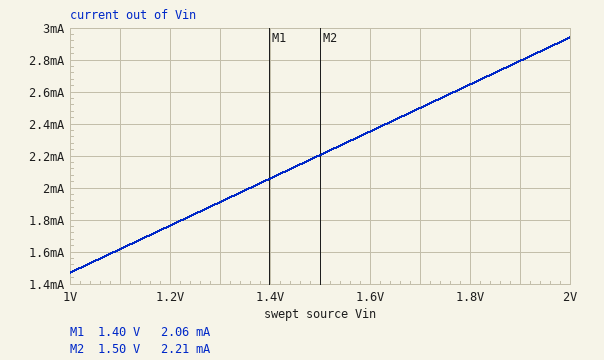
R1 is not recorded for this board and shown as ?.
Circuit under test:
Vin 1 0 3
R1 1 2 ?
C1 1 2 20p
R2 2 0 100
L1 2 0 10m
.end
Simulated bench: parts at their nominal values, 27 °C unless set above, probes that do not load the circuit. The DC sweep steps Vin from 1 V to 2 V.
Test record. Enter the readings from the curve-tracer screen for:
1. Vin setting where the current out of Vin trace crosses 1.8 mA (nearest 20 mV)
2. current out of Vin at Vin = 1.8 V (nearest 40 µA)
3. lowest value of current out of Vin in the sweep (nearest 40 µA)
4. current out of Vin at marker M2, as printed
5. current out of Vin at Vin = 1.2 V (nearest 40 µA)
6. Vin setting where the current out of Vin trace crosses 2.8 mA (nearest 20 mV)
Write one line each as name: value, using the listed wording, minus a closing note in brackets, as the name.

Vin setting where the current out of Vin trace crosses 1.8 mA: 1.22 V
current out of Vin at Vin = 1.8 V: 2.64 mA
lowest value of current out of Vin in the sweep: 1.48 mA
current out of Vin at marker M2, as printed: 2.21 mA
current out of Vin at Vin = 1.2 V: 1.76 mA
Vin setting where the current out of Vin trace crosses 2.8 mA: 1.90 V
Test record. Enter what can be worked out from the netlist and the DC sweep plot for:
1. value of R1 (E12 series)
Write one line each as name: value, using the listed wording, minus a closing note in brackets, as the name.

value of R1: 680 Ω
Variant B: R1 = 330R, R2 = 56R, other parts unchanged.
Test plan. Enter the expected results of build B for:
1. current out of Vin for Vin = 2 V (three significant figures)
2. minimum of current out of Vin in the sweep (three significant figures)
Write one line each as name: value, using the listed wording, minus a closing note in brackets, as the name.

current out of Vin for Vin = 2 V: 6.06 mA
minimum of current out of Vin in the sweep: 3.03 mA
